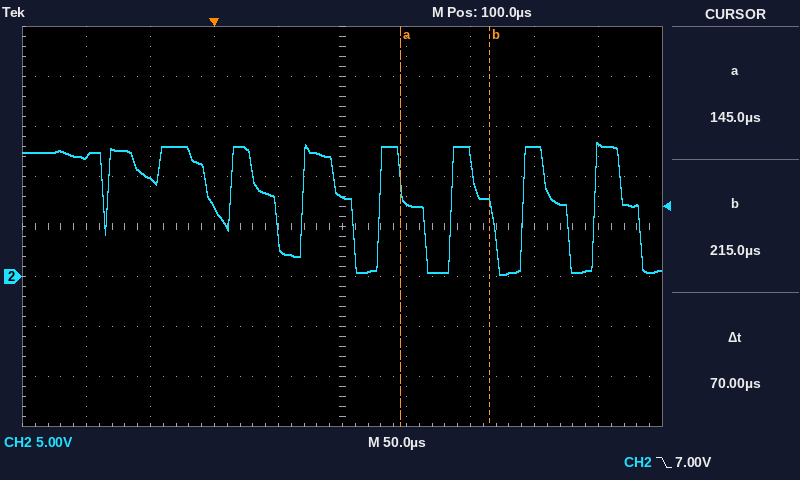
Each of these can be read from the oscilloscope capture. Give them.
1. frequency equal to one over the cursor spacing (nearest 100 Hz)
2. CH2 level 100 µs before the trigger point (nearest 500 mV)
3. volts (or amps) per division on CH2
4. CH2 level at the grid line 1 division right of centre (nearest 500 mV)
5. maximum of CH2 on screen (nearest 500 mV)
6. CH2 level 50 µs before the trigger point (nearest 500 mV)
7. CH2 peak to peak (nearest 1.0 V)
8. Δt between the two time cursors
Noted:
14.3 kHz
12.0 V
5 V
7.5 V
13.5 V
10.0 V
13.0 V
70 µs
